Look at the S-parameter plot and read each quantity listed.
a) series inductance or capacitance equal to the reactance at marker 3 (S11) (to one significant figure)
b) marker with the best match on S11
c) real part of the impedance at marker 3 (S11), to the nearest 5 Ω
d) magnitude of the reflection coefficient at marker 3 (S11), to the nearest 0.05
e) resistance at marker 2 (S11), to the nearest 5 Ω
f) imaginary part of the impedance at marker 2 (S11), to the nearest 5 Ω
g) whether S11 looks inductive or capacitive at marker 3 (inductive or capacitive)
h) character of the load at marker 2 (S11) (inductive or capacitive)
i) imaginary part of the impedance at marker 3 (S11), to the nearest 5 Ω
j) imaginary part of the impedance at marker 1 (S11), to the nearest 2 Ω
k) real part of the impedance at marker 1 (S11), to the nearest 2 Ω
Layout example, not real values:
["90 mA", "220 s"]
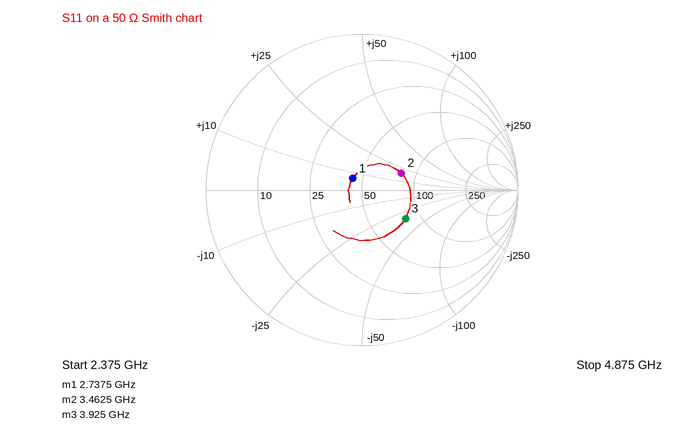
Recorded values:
["1 pF", "marker 1", "80 Ω", "0.35", "80 Ω", "+20 Ω", "capacitive", "inductive", "-35 Ω", "+6 Ω", "44 Ω"]
